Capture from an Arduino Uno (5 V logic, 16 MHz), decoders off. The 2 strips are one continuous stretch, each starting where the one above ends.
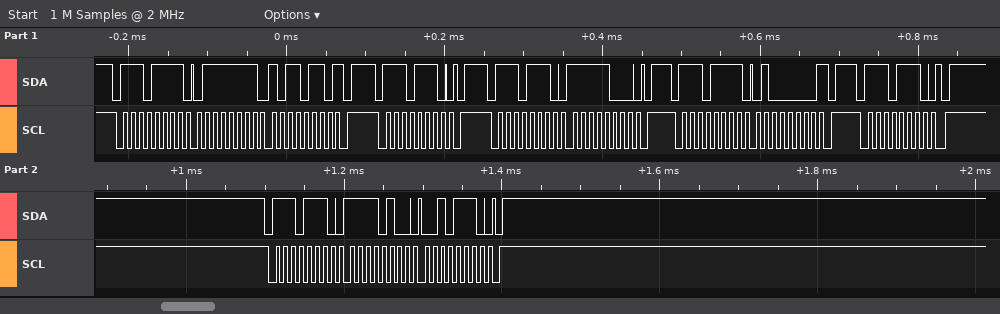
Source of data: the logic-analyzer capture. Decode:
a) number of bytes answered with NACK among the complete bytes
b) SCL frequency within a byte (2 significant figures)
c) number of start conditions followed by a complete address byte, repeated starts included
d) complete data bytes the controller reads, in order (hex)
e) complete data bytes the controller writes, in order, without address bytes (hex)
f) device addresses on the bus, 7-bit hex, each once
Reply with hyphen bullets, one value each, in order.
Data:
- 2
- 100 kHz
- 6
- 7F B6 40
- F8 F4 2E
- 0x77
